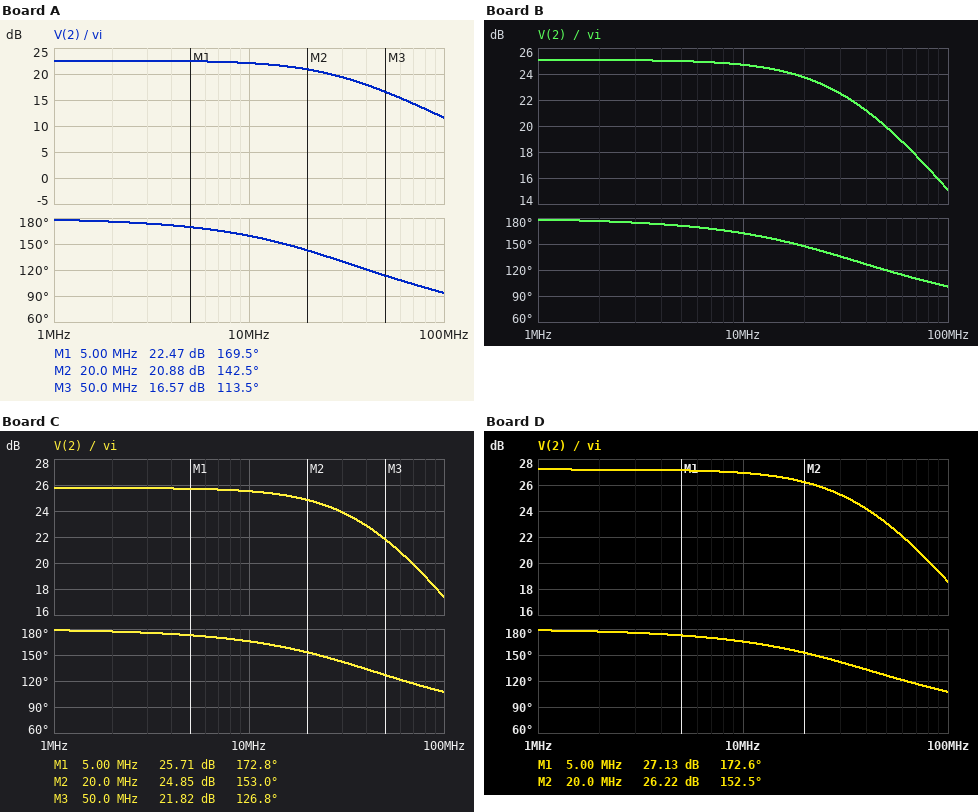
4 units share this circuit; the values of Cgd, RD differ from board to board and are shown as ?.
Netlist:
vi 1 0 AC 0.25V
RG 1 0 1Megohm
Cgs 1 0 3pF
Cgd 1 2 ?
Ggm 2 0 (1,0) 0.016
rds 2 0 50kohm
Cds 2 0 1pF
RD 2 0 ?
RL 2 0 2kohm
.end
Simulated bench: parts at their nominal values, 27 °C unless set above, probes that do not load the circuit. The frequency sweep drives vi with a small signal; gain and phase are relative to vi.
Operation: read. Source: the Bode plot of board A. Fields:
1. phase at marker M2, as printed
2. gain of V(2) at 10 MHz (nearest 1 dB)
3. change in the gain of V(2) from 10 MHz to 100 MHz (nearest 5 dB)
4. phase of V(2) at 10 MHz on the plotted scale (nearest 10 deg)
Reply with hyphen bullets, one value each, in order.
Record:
- 142.5 deg
- 22 dB
- -10 dB
- 160 deg
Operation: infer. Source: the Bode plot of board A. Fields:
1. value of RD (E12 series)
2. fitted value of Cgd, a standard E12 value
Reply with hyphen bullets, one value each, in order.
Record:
- 1.5 kΩ
- 5.6 pF
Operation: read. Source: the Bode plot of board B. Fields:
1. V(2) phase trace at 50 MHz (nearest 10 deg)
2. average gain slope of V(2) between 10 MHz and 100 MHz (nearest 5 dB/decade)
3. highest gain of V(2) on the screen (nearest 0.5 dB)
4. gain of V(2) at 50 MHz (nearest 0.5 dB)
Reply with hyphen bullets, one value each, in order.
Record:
- 120 deg
- -10 dB/decade
- 25.0 dB
- 20.0 dB
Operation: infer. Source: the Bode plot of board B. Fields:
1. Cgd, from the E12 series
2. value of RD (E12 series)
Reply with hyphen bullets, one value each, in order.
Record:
- 3.3 pF
- 2.7 kΩ
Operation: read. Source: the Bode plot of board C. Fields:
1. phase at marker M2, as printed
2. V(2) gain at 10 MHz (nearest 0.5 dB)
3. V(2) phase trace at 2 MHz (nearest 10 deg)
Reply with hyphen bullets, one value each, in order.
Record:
- 153.0 deg
- 25.5 dB
- 180 deg
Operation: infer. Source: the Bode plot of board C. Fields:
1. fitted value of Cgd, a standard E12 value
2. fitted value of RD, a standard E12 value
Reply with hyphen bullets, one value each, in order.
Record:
- 2.2 pF
- 3.3 kΩ
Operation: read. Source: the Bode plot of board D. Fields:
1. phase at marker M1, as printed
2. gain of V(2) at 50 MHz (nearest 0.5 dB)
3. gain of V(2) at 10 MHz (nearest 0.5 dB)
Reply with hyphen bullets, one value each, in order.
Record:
- 172.6 deg
- 23.0 dB
- 27.0 dB
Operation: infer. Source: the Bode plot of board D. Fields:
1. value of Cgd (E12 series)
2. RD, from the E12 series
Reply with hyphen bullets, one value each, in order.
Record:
- 1.8 pF
- 5.6 kΩ
